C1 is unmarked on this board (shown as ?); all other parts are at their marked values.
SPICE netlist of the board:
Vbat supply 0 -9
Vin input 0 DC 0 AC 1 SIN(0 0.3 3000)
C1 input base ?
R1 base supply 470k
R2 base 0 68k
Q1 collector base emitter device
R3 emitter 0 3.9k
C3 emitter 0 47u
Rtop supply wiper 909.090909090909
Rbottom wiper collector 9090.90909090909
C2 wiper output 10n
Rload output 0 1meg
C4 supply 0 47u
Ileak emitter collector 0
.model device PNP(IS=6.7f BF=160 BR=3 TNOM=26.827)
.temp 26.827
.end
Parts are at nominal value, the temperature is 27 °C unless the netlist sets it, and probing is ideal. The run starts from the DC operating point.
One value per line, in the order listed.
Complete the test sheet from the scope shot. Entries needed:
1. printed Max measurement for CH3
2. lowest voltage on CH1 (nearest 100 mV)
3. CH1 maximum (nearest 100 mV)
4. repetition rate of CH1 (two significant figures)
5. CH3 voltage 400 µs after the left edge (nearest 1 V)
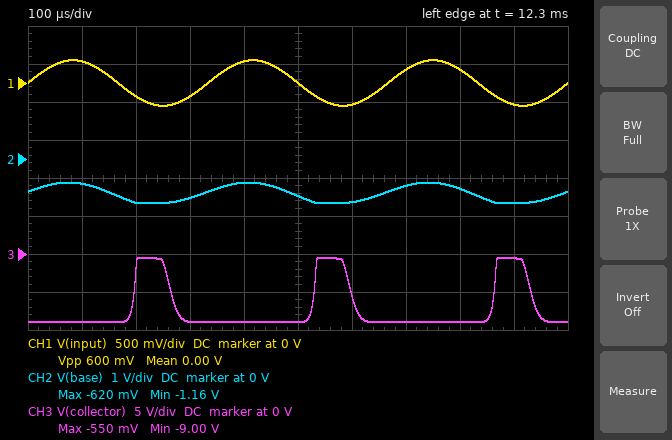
-550 mV
-300 mV
300 mV
3.0 kHz
-9 V
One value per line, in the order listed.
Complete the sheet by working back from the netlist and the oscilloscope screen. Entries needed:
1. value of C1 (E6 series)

10 nF
